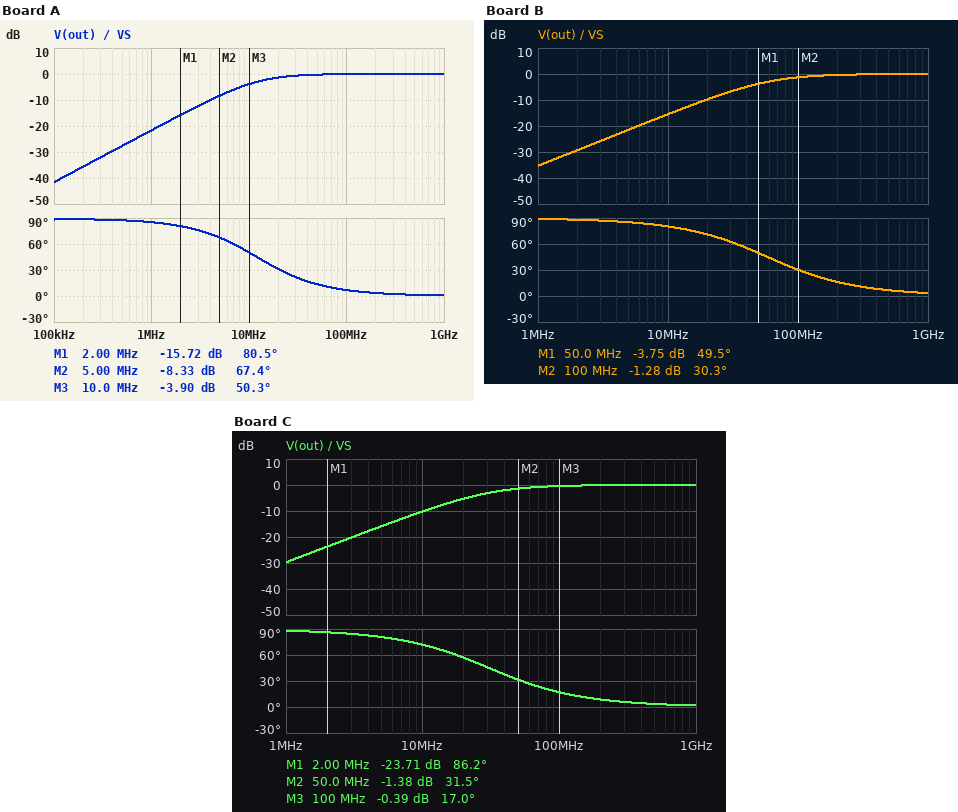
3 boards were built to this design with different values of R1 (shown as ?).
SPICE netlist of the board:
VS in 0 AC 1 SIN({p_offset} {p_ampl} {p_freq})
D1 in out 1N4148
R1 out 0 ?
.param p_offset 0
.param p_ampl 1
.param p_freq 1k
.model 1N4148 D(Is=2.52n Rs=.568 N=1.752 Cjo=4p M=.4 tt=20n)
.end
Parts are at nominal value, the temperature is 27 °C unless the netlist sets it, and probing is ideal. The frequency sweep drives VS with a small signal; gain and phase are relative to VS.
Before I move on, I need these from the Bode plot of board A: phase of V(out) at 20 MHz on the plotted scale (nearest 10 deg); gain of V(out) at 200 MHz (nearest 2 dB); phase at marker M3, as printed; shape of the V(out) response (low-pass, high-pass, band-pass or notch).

30 deg
0 dB
50.3 deg
high-pass
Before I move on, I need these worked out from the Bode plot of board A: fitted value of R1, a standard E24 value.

3.3 kΩ
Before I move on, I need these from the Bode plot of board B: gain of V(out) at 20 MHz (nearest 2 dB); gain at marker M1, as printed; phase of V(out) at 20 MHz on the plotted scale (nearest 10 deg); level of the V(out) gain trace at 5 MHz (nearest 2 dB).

-10 dB
-3.75 dB
70 deg
-22 dB
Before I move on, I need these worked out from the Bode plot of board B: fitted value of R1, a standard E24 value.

680 Ω
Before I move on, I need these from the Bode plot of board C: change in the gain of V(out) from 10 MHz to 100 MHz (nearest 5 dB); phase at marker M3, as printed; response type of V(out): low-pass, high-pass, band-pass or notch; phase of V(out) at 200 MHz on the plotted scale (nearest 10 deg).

10 dB
17.0 deg
high-pass
10 deg
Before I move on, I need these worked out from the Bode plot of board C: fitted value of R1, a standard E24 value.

1.3 kΩ
